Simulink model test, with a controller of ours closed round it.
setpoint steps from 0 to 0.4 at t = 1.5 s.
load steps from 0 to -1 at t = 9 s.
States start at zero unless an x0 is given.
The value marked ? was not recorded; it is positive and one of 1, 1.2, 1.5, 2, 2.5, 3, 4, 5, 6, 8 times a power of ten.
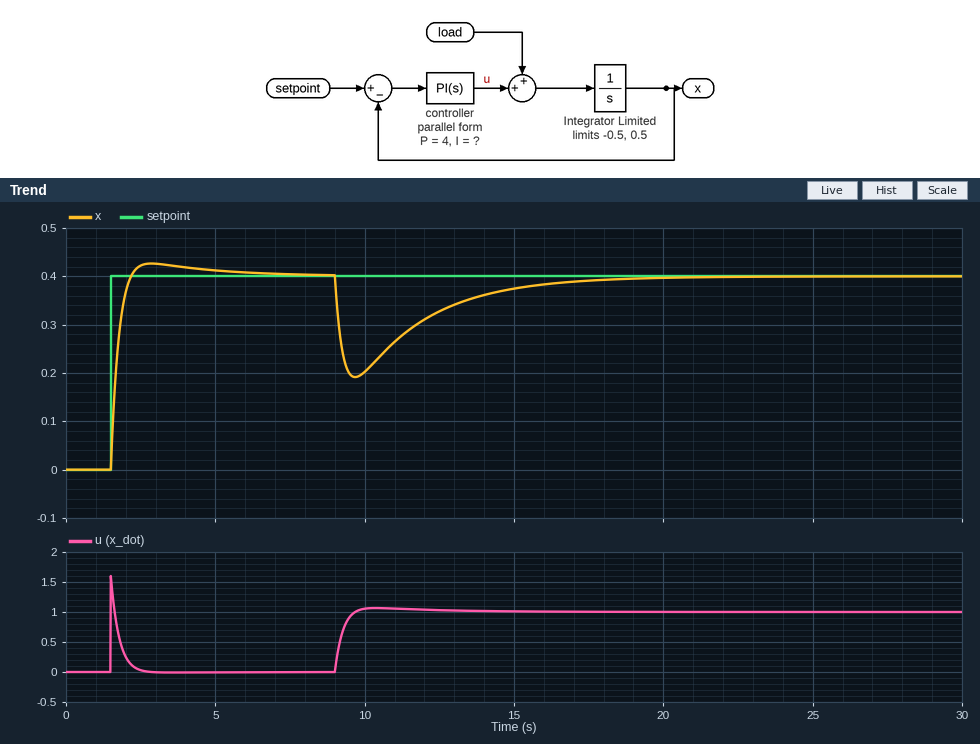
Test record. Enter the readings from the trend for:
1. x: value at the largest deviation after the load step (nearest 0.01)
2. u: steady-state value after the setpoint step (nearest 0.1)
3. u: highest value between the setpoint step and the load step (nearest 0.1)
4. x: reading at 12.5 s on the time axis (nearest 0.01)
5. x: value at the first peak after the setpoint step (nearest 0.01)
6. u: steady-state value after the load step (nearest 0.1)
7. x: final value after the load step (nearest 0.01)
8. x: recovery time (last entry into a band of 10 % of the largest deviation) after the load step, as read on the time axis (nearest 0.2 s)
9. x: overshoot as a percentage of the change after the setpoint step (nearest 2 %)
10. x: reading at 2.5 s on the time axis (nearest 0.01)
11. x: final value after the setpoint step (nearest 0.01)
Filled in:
0.19
0.0
1.6
0.33
0.43
1.0
0.40
15.4 s
6 %
0.42
0.40
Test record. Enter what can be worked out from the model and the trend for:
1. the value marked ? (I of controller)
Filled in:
1.5
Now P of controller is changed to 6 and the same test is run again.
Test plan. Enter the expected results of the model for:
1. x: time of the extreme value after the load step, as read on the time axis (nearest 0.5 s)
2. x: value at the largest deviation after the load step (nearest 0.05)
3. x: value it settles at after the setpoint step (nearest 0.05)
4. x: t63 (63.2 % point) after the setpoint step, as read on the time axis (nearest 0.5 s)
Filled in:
9.5 s
0.25
0.40
1.5 s
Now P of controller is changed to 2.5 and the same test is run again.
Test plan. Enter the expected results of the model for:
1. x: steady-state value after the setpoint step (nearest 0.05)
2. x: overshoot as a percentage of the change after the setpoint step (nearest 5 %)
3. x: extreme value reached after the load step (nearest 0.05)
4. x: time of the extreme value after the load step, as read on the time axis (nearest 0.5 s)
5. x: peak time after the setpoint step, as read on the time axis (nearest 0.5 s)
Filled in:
0.40
15 %
0.10
10.0 s
3.0 s
